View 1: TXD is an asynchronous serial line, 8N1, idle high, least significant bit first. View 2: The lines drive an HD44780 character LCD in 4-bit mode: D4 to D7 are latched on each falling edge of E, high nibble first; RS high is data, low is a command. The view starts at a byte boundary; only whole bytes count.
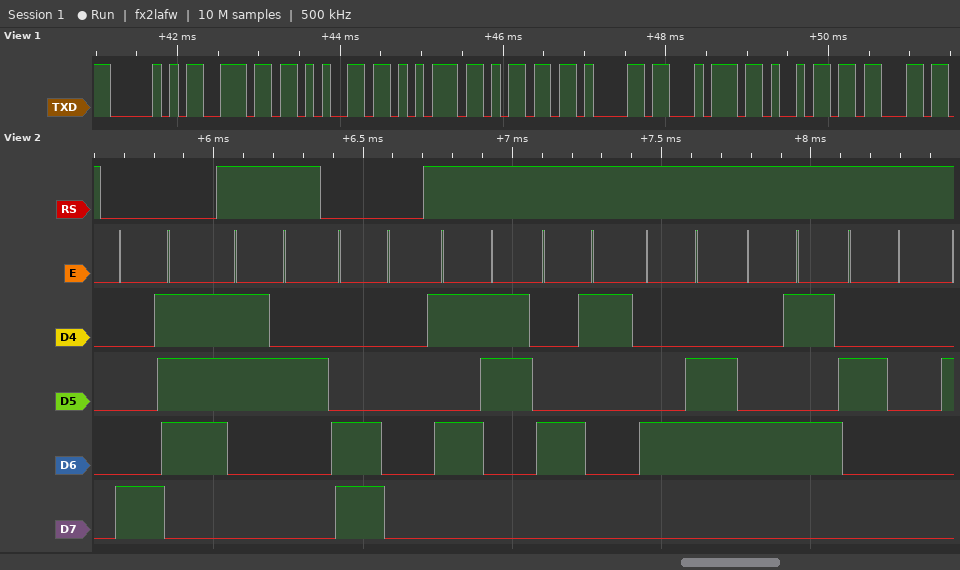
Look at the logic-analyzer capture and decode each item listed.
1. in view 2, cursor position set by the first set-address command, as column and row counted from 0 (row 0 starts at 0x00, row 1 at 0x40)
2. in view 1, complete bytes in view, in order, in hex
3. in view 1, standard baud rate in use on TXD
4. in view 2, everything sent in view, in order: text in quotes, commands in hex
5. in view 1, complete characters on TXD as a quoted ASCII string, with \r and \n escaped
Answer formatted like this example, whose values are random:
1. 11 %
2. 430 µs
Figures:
1. column 7, row 0
2. 0x50 0x6E 0x65 0x75 0x6D 0x61 0x74 0x69 0x63
3. 9600 baud
4. 0x87 "2" 0xC0 "SAFE "
5. "Pneumatic"
